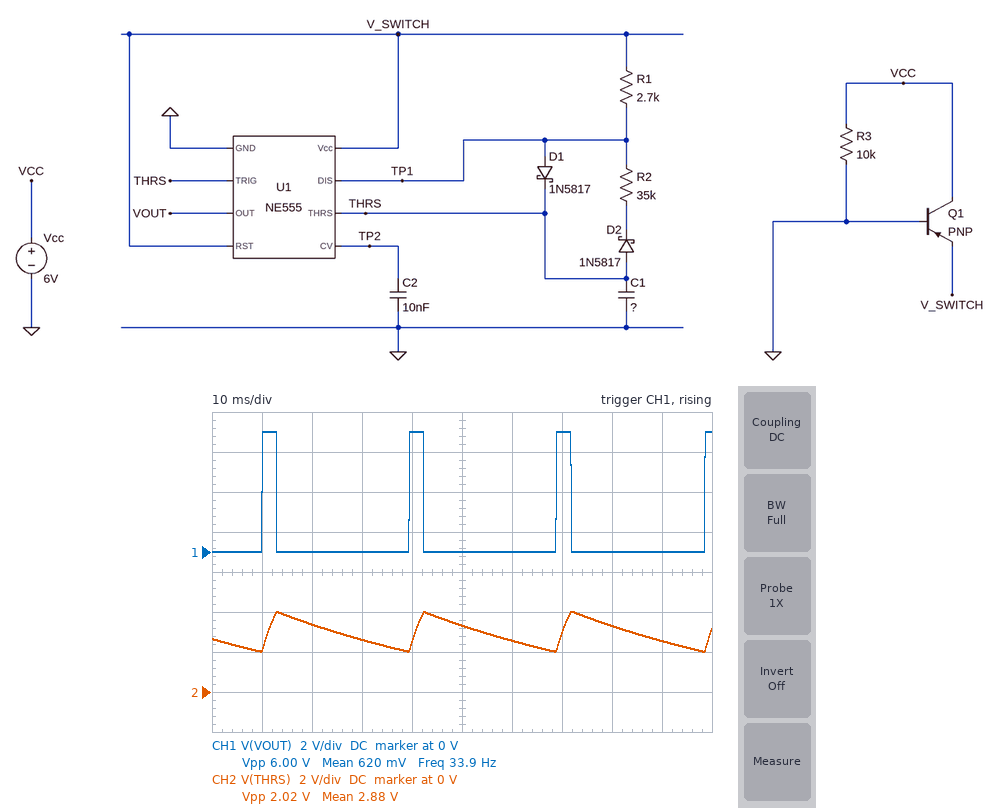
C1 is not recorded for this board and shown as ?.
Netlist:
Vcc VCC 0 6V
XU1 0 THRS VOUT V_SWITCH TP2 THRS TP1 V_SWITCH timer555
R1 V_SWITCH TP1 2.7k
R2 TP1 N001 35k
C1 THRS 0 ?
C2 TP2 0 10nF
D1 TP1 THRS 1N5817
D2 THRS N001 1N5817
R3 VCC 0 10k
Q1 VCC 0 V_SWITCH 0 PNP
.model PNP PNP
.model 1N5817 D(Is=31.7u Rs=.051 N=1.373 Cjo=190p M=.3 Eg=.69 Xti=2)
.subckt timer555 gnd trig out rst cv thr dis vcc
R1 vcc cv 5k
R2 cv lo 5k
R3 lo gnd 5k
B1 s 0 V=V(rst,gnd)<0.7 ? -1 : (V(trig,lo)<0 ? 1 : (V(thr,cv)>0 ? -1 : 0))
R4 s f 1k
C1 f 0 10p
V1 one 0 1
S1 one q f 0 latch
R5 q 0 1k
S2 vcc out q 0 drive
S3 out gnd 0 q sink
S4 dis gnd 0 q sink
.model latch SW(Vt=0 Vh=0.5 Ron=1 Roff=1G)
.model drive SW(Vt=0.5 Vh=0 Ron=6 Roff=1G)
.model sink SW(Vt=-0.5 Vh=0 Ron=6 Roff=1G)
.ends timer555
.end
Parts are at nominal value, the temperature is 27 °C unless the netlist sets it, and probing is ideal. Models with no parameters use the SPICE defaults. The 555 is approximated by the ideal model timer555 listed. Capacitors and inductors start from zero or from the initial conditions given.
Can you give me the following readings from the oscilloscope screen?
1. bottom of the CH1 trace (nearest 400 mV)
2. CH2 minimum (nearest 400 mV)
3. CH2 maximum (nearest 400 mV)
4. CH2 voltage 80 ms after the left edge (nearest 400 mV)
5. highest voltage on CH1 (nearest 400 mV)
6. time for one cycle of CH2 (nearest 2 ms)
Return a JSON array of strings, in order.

["0 V", "2.0 V", "4.0 V", "3.2 V", "6.0 V", "30 ms"]
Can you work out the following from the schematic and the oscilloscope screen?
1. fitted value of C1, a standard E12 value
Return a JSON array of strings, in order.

["1.5 µF"]
